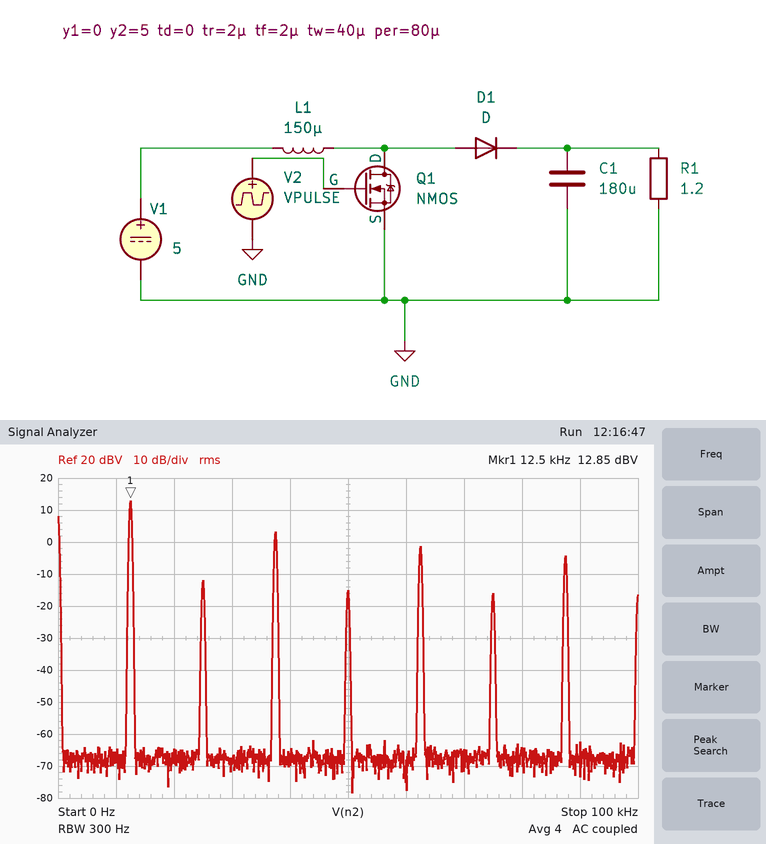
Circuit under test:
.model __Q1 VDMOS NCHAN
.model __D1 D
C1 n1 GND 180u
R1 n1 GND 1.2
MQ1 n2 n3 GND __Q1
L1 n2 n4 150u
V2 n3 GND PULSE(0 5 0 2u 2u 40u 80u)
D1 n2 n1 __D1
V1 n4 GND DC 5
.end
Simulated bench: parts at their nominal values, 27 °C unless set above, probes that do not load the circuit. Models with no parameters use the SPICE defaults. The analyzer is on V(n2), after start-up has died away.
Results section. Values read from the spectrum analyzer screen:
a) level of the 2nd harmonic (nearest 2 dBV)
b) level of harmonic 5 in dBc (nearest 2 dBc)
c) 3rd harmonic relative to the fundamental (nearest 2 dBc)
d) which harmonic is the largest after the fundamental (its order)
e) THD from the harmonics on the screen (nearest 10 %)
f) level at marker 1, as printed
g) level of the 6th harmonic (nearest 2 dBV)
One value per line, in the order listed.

-12 dBV
-14 dBc
-10 dBc
3
40 %
12.85 dBV
-16 dBV
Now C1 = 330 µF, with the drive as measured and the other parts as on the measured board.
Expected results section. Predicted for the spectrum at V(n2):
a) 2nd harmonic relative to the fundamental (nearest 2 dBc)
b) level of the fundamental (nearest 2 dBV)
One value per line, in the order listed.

-28 dBc
12 dBV
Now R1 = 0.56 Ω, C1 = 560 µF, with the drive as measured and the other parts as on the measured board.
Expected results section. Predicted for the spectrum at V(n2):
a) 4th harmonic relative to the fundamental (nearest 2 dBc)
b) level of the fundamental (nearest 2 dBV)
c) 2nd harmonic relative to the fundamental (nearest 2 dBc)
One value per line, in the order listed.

-32 dBc
12 dBV
-28 dBc
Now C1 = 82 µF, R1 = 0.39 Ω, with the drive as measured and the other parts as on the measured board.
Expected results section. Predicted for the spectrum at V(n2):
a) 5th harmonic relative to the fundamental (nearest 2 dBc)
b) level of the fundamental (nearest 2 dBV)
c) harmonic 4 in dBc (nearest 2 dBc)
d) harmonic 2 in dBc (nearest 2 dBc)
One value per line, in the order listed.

-16 dBc
12 dBV
-18 dBc
-12 dBc
